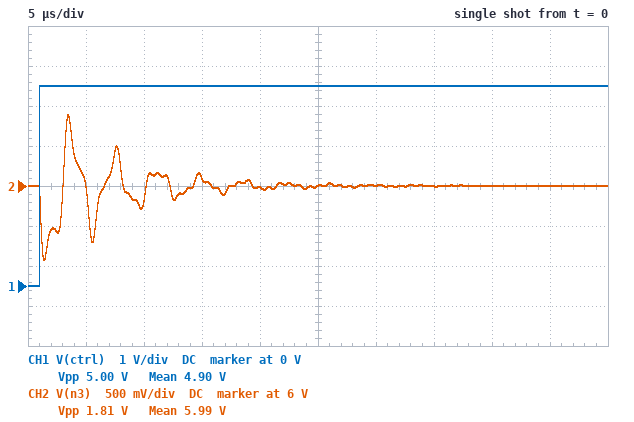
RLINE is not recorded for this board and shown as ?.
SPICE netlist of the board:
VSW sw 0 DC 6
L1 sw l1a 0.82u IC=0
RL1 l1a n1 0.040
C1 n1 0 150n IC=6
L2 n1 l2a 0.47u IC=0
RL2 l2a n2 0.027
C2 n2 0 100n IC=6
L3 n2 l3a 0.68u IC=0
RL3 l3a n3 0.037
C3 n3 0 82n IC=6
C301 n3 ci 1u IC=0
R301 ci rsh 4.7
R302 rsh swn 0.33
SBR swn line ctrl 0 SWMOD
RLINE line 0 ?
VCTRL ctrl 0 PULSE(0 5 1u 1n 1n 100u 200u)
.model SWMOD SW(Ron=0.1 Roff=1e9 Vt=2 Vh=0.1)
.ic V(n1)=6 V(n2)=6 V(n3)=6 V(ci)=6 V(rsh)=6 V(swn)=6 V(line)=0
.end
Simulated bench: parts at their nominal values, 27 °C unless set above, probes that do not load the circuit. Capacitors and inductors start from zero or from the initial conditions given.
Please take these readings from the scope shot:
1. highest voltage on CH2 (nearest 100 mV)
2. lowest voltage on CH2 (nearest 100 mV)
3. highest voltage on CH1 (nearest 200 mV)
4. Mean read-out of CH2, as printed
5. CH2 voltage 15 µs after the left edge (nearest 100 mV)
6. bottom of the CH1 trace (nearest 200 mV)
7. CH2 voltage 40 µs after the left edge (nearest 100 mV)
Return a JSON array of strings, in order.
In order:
["6.9 V", "5.1 V", "5.0 V", "5.99 V", "6.1 V", "0 V", "6.0 V"]
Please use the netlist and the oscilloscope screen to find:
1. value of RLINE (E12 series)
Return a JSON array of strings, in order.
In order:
["12 Ω"]
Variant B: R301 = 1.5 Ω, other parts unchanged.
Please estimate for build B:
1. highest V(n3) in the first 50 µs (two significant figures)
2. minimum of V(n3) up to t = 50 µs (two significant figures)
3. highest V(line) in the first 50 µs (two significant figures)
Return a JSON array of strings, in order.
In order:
["7.0 V", "4.9 V", "5.3 V"]
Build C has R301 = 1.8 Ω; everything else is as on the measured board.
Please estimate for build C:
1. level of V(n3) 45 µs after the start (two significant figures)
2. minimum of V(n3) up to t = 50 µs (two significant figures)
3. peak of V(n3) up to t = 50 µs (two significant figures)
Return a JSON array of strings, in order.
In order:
["6.0 V", "4.9 V", "7.0 V"]
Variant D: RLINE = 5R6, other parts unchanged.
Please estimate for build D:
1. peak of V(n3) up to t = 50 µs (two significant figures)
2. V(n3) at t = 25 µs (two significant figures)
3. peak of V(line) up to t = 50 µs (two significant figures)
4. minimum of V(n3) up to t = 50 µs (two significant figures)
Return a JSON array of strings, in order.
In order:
["7.2 V", "6.0 V", "3.2 V", "4.6 V"]
